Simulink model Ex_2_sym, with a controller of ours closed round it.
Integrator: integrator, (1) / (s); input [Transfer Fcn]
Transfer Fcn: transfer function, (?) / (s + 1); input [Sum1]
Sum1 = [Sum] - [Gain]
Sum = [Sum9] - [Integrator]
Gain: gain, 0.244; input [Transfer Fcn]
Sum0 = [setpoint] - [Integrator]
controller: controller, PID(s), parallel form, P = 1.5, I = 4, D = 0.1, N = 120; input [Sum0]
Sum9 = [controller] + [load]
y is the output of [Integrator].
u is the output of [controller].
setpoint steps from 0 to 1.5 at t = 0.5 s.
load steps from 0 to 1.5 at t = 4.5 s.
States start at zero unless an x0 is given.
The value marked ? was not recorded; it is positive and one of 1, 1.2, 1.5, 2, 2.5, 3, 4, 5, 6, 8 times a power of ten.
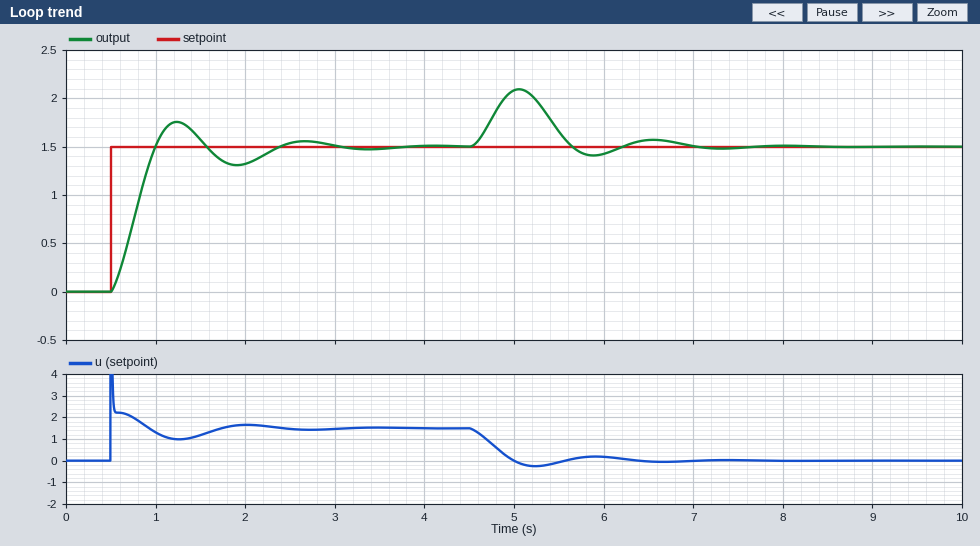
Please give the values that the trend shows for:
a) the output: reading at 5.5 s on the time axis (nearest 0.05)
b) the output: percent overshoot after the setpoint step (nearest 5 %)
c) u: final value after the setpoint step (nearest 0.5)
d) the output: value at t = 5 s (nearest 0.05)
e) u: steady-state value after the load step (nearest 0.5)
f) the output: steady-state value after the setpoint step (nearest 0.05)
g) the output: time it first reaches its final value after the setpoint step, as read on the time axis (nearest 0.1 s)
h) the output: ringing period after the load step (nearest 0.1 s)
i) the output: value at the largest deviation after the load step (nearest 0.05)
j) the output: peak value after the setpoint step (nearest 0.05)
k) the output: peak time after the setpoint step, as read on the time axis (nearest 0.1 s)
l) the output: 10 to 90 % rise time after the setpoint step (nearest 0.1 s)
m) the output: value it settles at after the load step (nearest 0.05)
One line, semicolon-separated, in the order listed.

1.65; 15 %; 1.5; 2.10; 0.0; 1.50; 1.0 s; 1.5 s; 2.10; 1.75; 1.2 s; 0.4 s; 1.50
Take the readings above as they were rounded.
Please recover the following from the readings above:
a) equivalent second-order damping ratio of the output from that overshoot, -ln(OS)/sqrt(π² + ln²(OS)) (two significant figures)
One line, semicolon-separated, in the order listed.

0.52
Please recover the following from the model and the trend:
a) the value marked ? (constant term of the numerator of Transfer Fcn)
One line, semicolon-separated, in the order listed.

10
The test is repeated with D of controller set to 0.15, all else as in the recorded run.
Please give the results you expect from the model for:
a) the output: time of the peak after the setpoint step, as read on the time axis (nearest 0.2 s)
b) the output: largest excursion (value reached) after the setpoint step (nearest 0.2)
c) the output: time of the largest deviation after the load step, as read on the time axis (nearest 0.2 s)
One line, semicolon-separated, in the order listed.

1.2 s; 1.6; 5.0 s
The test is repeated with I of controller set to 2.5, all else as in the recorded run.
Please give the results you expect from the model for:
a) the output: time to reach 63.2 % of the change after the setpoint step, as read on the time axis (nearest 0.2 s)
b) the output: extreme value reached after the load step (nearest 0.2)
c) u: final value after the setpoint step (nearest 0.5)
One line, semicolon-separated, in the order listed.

0.8 s; 2.2; 1.5
